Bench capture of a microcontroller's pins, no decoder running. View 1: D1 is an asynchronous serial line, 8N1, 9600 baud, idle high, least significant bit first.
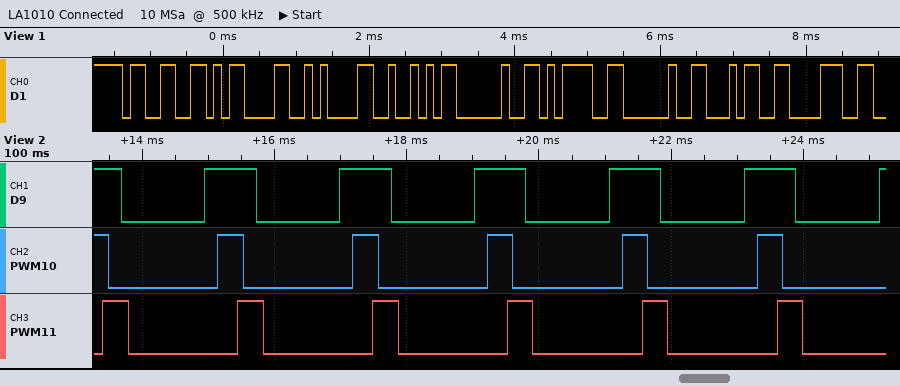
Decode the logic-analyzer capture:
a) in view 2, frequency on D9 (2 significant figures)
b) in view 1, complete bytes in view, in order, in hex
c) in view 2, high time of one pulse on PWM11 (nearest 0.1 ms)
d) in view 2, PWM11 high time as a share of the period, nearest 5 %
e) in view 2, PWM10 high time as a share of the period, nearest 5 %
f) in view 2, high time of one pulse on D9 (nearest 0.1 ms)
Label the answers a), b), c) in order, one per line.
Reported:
a) 490 Hz
b) 33 0D 0A 52 20 3D 20 34 38
c) 0.4 ms
d) 20 %
e) 20 %
f) 0.8 ms
